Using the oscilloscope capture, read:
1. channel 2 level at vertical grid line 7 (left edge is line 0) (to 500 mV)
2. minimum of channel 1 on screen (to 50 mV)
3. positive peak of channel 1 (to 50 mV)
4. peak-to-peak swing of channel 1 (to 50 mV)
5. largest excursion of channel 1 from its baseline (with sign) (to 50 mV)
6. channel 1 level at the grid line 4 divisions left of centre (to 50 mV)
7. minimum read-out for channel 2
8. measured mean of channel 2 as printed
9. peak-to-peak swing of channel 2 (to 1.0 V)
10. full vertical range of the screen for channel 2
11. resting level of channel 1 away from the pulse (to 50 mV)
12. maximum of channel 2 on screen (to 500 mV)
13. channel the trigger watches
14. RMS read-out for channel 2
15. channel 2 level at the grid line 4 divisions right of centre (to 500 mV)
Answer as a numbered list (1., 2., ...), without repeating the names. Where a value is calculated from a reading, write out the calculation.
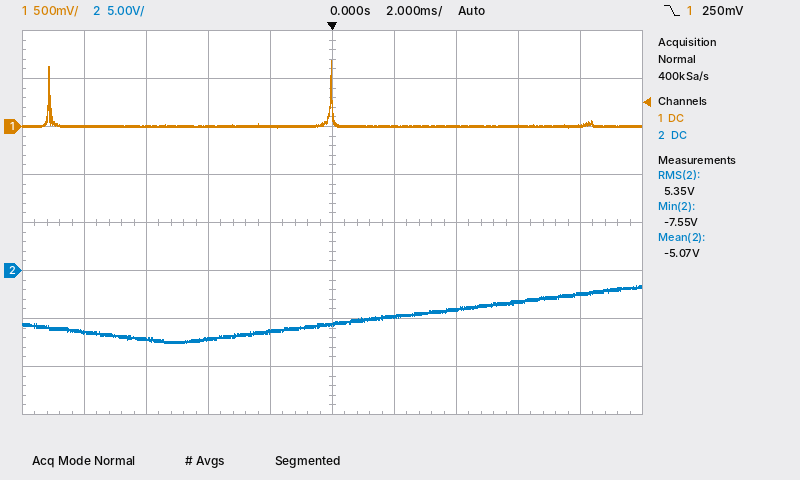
1. -4.0 V
2. 0 mV
3. 700 mV
4. 700 mV − (0 mV) = 700 mV
5. 700 mV − (0 mV) = +700 mV
6. 0 mV
7. -7.55 V
8. -5.07 V
9. 6.0 V
10. 40 V
11. 0 mV
12. -1.5 V
13. channel 1
14. 5.35 V
15. -2.5 V
